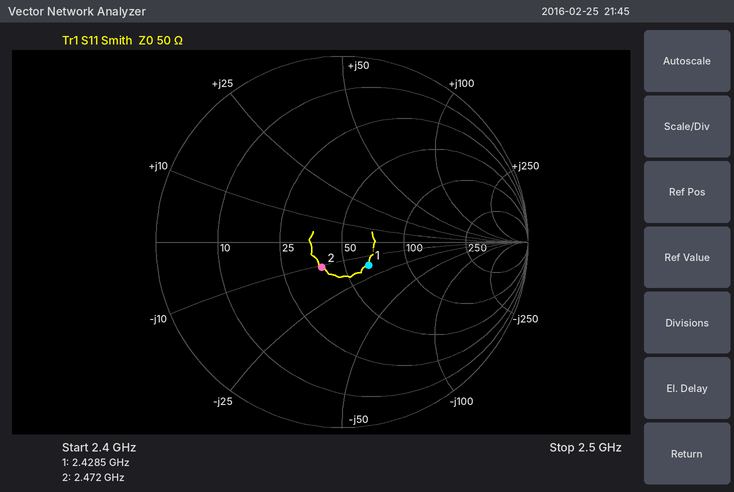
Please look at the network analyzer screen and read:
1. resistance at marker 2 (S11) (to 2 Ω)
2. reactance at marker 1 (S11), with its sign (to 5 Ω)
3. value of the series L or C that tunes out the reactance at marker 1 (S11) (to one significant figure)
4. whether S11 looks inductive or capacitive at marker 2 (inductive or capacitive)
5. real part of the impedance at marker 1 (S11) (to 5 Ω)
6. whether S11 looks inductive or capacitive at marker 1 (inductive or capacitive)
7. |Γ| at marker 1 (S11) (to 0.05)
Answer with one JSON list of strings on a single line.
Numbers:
["38 Ω", "-15 Ω", "1 nH", "capacitive", "65 Ω", "capacitive", "0.20"]
